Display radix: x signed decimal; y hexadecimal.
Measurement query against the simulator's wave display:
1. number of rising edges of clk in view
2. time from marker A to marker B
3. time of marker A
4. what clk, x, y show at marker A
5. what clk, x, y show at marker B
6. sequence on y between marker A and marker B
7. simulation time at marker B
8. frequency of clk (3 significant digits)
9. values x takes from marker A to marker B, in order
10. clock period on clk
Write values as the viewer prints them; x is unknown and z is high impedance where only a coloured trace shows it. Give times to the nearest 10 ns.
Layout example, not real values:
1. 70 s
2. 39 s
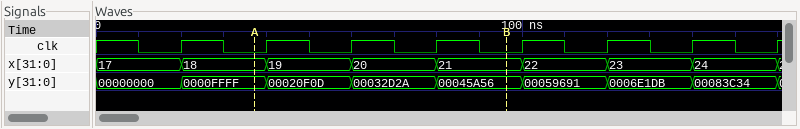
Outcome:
1. 8
2. 60 ns
3. 40 ns
4. clk=0, x=18, y=0000FFFF
5. clk=0, x=21, y=00045A56
6. 0000FFFF, 00020F0D, 00032D2A, 00045A56
7. 100 ns
8. 50.0 MHz
9. 18, 19, 20, 21
10. 20 ns
